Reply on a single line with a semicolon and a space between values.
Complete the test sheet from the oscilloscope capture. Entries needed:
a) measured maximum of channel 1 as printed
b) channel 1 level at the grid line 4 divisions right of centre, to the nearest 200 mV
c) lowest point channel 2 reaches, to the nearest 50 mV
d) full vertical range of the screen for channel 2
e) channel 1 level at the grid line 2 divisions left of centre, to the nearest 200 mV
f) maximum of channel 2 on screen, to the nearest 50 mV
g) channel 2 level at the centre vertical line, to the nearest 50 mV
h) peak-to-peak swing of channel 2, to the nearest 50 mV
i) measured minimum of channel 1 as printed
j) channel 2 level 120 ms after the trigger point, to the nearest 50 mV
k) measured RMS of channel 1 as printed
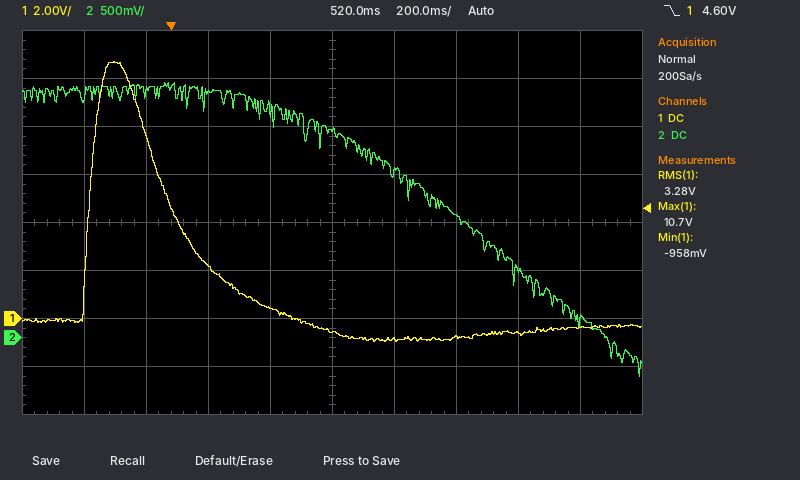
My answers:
10.7 V; -400 mV; -400 mV; 4 V; 2.2 V; 2.65 V; 2.15 V; 3.05 V; -958 mV; 2.55 V; 3.28 V
